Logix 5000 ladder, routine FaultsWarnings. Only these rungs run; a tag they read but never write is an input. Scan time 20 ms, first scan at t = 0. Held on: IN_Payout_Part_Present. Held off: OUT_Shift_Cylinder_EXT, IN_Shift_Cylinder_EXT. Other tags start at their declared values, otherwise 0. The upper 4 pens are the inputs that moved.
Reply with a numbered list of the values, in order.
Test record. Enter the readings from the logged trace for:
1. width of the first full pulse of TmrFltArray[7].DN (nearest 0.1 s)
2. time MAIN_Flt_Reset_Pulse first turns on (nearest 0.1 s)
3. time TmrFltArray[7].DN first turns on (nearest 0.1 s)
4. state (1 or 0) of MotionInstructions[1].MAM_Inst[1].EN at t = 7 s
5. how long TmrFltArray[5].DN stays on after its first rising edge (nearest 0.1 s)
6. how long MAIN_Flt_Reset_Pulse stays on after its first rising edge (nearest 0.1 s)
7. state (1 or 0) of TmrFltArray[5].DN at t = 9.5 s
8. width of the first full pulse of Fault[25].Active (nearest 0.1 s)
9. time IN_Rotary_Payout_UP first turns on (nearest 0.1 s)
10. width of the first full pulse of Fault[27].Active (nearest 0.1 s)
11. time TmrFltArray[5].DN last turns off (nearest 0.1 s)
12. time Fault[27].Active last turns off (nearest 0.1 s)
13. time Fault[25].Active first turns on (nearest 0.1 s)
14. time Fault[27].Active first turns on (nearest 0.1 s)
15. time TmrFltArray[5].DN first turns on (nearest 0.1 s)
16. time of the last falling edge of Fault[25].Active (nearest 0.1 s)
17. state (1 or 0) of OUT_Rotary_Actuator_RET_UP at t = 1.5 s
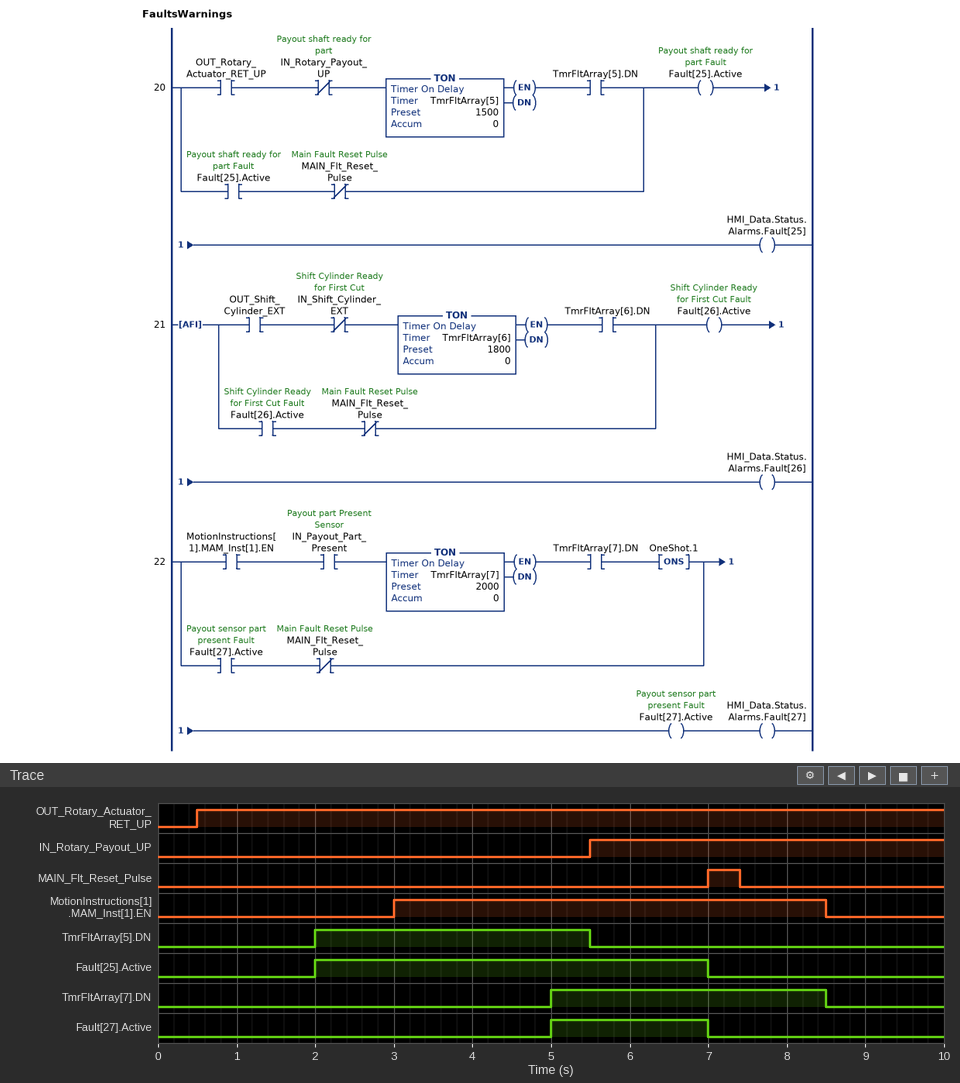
1. 3.5 s
2. 7.0 s
3. 5.0 s
4. 1
5. 3.5 s
6. 0.4 s
7. 0
8. 5.0 s
9. 5.5 s
10. 2.0 s
11. 5.5 s
12. 7.0 s
13. 2.0 s
14. 5.0 s
15. 2.0 s
16. 7.0 s
17. 1
